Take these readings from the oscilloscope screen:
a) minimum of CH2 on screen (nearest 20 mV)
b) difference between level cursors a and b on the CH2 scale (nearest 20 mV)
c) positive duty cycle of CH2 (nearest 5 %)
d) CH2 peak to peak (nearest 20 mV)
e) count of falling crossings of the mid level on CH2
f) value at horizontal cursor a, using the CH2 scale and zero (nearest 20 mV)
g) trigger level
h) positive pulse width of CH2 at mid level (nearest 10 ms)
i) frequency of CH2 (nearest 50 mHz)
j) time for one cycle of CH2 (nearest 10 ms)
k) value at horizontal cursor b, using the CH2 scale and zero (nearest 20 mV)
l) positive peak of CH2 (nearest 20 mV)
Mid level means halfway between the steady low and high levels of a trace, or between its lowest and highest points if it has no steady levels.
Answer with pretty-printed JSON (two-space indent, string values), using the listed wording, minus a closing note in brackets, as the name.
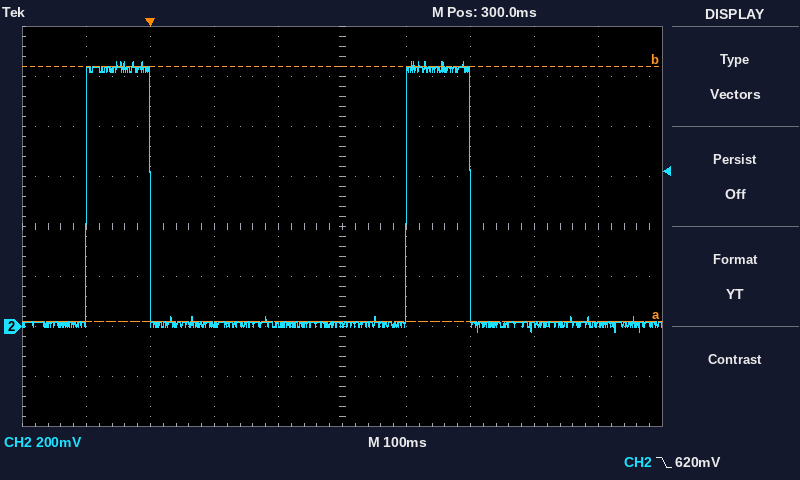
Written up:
{
  "minimum of CH2 on screen": "-20 mV",
  "difference between level cursors a and b on the CH2 scale": "1.02 V",
  "positive duty cycle of CH2": "20 %",
  "CH2 peak to peak": "1.08 V",
  "count of falling crossings of the mid level on CH2": "2",
  "value at horizontal cursor a, using the CH2 scale and zero": "20 mV",
  "trigger level": "620 mV",
  "positive pulse width of CH2 at mid level": "100 ms",
  "frequency of CH2": "2.00 Hz",
  "time for one cycle of CH2": "500 ms",
  "value at horizontal cursor b, using the CH2 scale and zero": "1.04 V",
  "positive peak of CH2": "1.06 V"
}
